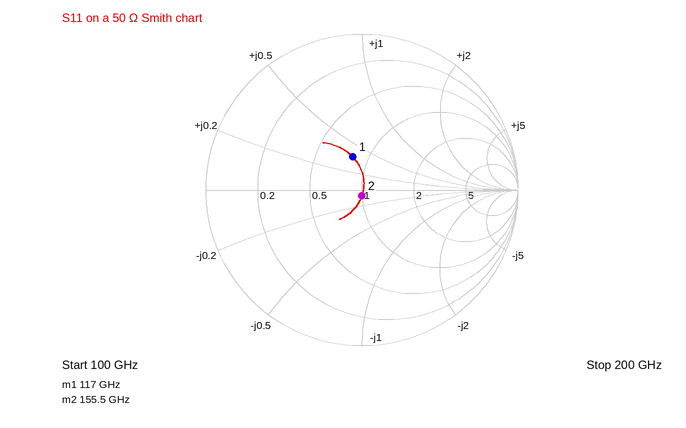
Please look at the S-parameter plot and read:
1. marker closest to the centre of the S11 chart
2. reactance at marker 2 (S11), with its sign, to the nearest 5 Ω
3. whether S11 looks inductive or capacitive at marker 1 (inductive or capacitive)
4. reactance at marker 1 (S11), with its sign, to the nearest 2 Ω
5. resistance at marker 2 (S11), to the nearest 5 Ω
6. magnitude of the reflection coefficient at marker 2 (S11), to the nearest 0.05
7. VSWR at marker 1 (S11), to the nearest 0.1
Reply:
marker 2
-5 Ω
inductive
+18 Ω
50 Ω
0.05
1.6
